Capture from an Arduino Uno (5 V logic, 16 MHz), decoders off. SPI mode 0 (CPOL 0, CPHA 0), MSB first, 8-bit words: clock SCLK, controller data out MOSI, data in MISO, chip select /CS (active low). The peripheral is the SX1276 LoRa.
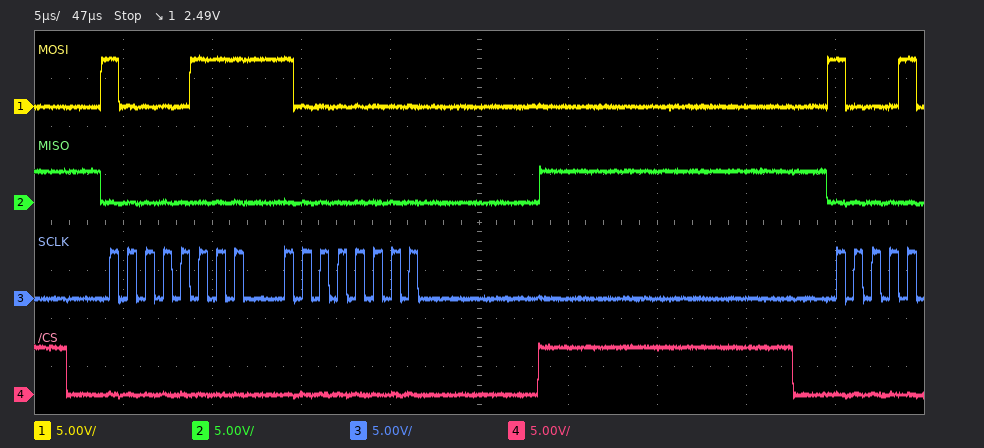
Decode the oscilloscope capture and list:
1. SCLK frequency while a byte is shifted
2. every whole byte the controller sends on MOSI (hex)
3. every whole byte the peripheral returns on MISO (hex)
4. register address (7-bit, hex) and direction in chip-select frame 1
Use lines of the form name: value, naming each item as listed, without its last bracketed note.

SCLK frequency while a byte is shifted: 1 MHz
every whole byte the controller sends on MOSI: 87 80
every whole byte the peripheral returns on MISO: 00 00
register address (7-bit, hex) and direction in chip-select frame 1: 0x07 write
